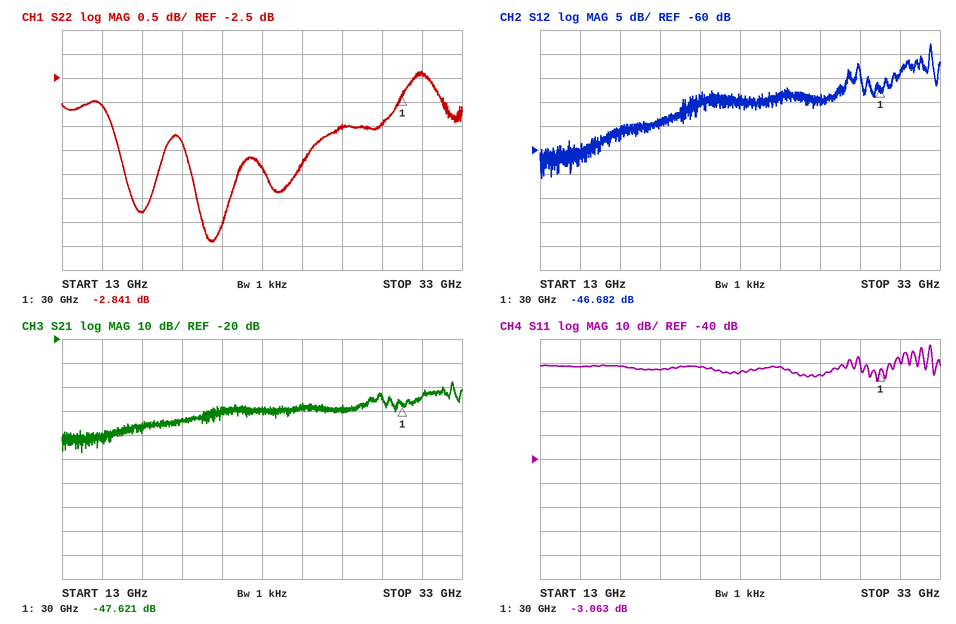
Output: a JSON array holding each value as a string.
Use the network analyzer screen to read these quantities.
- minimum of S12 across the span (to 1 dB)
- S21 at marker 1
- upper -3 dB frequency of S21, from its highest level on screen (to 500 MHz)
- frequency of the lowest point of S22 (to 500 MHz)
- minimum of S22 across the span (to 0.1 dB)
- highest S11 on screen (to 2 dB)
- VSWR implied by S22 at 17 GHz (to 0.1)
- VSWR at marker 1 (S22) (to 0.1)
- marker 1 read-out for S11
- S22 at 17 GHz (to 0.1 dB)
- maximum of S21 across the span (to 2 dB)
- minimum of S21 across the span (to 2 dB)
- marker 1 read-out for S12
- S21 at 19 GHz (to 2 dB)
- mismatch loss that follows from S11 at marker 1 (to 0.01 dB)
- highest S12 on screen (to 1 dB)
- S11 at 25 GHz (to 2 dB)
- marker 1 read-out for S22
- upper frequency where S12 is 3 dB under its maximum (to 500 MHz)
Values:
["-66 dB", "-47.621 dB", "32.5 GHz", "20.5 GHz", "-5.9 dB", "8 dB", "3.4", "6.2", "-3.063 dB", "-5.3 dB", "-38 dB", "-68 dB", "-46.682 dB", "-54 dB", "2.96 dB", "-38 dB", "-2 dB", "-2.841 dB", "32.5 GHz"]
